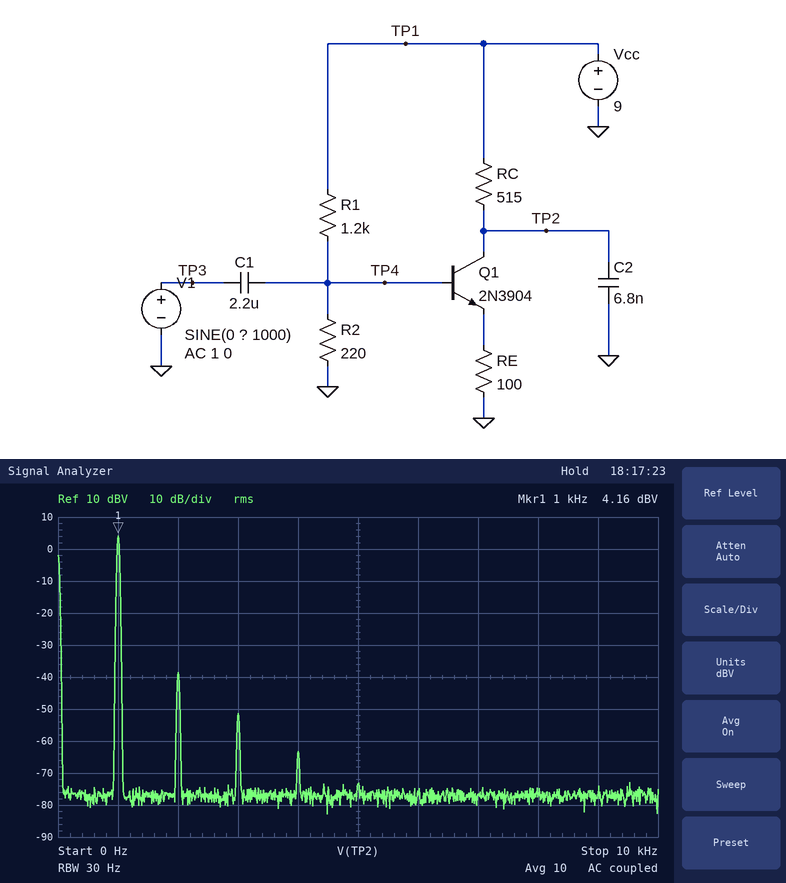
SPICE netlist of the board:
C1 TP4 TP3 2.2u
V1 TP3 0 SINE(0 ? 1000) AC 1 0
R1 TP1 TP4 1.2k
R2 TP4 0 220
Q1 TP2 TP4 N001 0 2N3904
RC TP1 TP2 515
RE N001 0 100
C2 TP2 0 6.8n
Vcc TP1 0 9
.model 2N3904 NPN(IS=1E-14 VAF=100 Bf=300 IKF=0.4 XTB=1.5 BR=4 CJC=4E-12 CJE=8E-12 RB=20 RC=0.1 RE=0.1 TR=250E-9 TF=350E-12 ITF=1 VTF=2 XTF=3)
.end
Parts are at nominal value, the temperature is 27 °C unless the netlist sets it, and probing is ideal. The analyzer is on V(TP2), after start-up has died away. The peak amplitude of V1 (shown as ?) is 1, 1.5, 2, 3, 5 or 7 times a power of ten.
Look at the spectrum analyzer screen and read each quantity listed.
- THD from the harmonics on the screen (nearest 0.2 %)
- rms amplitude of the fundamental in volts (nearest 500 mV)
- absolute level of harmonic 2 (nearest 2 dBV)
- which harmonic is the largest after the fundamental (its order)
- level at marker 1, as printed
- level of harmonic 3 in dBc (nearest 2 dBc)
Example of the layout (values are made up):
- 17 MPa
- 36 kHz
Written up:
- 0.8 %
- 1.5 V
- -38 dBV
- 2
- 4.16 dBV
- -56 dBc
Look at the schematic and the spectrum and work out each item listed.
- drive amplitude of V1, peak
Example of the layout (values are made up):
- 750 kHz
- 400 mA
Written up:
- 500 mV
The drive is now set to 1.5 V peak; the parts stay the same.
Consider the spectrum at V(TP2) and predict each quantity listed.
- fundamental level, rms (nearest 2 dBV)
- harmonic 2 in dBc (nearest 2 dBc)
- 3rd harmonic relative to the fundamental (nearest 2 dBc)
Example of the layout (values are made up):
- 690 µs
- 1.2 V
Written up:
- 10 dBV
- -22 dBc
- -14 dBc
